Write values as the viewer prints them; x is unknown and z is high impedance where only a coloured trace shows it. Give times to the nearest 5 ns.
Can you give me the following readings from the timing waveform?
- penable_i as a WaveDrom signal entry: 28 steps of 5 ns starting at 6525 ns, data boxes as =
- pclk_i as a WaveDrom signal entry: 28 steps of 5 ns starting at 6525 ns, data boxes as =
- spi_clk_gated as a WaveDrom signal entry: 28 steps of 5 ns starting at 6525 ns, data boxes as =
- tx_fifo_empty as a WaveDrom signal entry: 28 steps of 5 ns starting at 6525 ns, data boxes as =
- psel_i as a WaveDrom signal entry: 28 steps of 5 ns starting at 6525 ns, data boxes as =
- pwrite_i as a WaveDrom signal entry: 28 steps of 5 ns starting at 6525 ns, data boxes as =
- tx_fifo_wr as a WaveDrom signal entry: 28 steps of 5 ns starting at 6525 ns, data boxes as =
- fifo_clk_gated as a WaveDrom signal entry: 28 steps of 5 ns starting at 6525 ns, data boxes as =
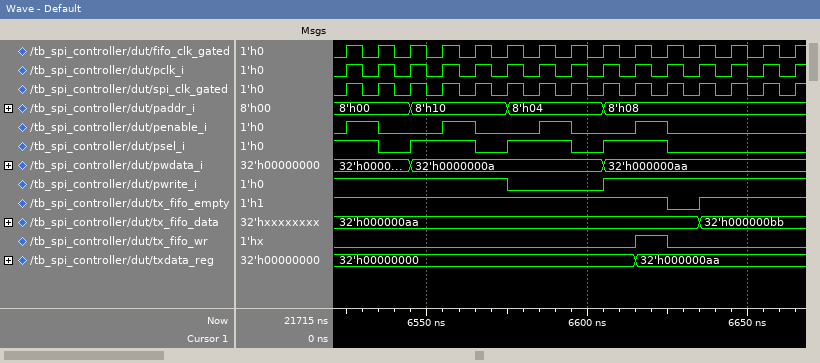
{name: 'penable_i', wave: '1.0...1.0...1.0...1.0.......'}
{name: 'pclk_i', wave: '1010101010101010101010101010'}
{name: 'spi_clk_gated', wave: '1010101010101010101010101010'}
{name: 'tx_fifo_empty', wave: '1...................0.1.....'}
{name: 'psel_i', wave: '1.0.1...0.1...0.1...0.......'}
{name: 'pwrite_i', wave: '1.........0.....1...........'}
{name: 'tx_fifo_wr', wave: '0.................1.0.......'}
{name: 'fifo_clk_gated', wave: '1010101010101010101010101010'}
